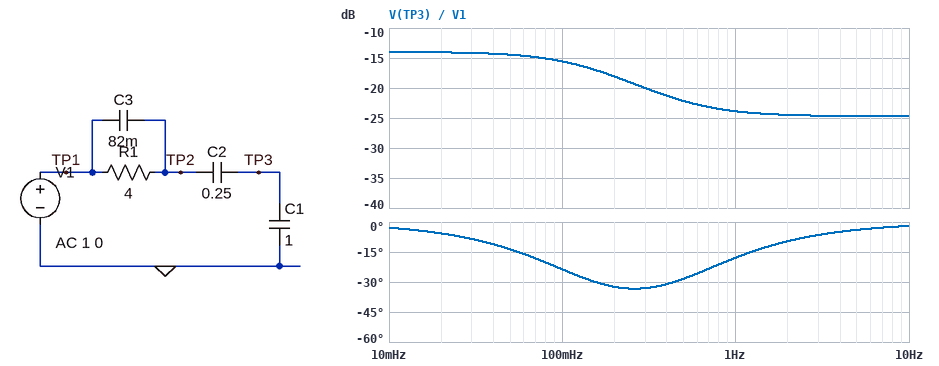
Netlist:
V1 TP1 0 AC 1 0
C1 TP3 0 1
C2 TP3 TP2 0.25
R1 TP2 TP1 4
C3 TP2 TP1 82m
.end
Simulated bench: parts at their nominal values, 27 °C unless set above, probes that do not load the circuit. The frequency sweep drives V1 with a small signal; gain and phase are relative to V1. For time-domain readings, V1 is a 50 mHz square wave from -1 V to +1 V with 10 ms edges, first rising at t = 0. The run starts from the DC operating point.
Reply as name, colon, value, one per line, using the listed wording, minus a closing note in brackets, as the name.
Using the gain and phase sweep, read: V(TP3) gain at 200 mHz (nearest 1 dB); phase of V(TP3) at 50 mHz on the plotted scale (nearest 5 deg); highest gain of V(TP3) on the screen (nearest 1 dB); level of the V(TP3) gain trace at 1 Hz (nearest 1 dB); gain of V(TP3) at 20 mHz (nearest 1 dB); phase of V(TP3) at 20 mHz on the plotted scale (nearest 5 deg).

V(TP3) gain at 200 mHz: -18 dB
phase of V(TP3) at 50 mHz on the plotted scale: -15 deg
highest gain of V(TP3) on the screen: -14 dB
level of the V(TP3) gain trace at 1 Hz: -24 dB
gain of V(TP3) at 20 mHz: -14 dB
phase of V(TP3) at 20 mHz on the plotted scale: -5 deg
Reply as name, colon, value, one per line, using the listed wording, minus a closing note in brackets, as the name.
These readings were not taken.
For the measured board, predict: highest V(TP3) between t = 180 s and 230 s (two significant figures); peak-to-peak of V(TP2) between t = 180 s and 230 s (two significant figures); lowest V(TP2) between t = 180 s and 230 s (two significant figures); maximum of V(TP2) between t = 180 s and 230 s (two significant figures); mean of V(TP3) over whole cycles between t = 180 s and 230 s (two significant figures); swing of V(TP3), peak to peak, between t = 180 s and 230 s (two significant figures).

highest V(TP3) between t = 180 s and 230 s: 400 mV
peak-to-peak of V(TP2) between t = 180 s and 230 s: 2.0 V
lowest V(TP2) between t = 180 s and 230 s: -1.0 V
maximum of V(TP2) between t = 180 s and 230 s: 1.0 V
mean of V(TP3) over whole cycles between t = 180 s and 230 s: 200 mV
swing of V(TP3), peak to peak, between t = 180 s and 230 s: 400 mV
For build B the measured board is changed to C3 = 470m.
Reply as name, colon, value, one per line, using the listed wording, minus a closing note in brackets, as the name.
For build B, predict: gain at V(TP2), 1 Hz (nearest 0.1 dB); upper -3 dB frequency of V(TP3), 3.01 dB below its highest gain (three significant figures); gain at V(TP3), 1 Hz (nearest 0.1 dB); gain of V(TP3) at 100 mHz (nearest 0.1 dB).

gain at V(TP2), 1 Hz: -3.1 dB
upper -3 dB frequency of V(TP3), 3.01 dB below its highest gain: 472 mHz
gain at V(TP3), 1 Hz: -17.0 dB
gain of V(TP3) at 100 mHz: -16.0 dB
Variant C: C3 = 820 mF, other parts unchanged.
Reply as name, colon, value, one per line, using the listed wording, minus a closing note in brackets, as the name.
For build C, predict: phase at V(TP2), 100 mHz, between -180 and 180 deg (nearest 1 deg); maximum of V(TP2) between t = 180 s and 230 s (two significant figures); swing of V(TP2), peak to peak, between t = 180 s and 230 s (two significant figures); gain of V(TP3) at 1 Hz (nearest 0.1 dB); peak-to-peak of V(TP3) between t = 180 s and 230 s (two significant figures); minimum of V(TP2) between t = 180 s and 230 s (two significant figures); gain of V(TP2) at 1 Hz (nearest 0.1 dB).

phase at V(TP2), 100 mHz, between -180 and 180 deg: -5 deg
maximum of V(TP2) between t = 180 s and 230 s: 970 mV
swing of V(TP2), peak to peak, between t = 180 s and 230 s: 1.9 V
gain of V(TP3) at 1 Hz: -15.9 dB
peak-to-peak of V(TP3) between t = 180 s and 230 s: 390 mV
minimum of V(TP2) between t = 180 s and 230 s: -970 mV
gain of V(TP2) at 1 Hz: -1.9 dB
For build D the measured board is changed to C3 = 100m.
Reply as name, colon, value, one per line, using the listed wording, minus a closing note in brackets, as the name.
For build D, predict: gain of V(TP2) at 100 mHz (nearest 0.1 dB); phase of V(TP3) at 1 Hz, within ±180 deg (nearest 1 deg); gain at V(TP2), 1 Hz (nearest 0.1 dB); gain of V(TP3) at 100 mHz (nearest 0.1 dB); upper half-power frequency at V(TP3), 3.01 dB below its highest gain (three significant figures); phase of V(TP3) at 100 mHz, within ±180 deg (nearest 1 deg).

gain of V(TP2) at 100 mHz: -1.7 dB
phase of V(TP3) at 1 Hz, within ±180 deg: -14 deg
gain at V(TP2), 1 Hz: -9.0 dB
gain of V(TP3) at 100 mHz: -15.7 dB
upper half-power frequency at V(TP3), 3.01 dB below its highest gain: 150 mHz
phase of V(TP3) at 100 mHz, within ±180 deg: -23 deg
